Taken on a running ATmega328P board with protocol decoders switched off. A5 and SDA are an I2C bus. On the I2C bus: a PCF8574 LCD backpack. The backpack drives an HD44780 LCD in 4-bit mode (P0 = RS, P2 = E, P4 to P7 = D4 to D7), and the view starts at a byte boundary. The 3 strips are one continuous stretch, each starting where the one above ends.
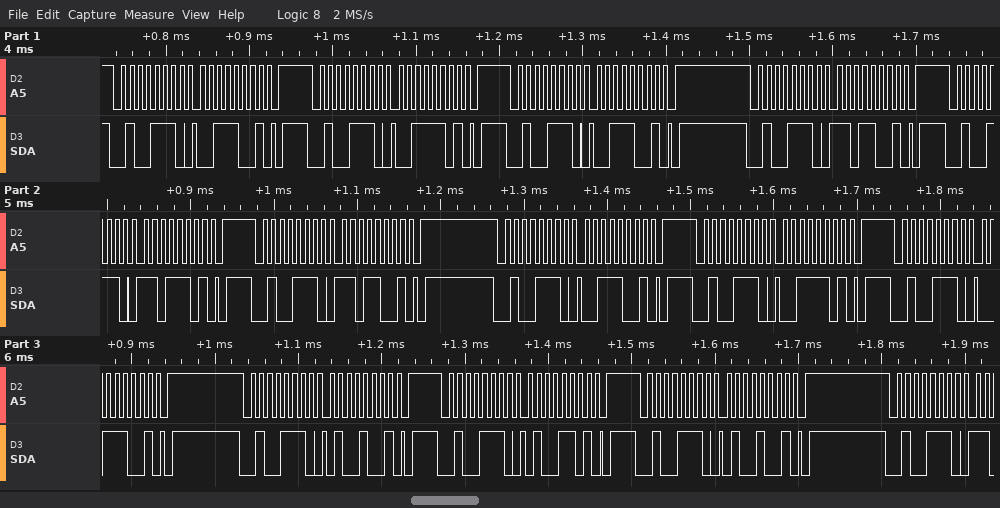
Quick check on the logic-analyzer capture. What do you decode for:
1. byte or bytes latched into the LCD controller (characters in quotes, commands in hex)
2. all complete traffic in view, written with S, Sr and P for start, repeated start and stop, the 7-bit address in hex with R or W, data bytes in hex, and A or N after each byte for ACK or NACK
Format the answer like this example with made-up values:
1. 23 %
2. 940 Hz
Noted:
1. '=' '4'
2. S 27W A 39 A P S 27W A 3D A P S 27W A 39 A P S 27W A D9 A P S 27W A DD A P S 27W A D9 A P S 27W A 39 A P S 27W A 3D A P S 27W A 39 A P S 27W A 49 A P S 27W A 4D A P S 27W A 49 A P S 27W A
